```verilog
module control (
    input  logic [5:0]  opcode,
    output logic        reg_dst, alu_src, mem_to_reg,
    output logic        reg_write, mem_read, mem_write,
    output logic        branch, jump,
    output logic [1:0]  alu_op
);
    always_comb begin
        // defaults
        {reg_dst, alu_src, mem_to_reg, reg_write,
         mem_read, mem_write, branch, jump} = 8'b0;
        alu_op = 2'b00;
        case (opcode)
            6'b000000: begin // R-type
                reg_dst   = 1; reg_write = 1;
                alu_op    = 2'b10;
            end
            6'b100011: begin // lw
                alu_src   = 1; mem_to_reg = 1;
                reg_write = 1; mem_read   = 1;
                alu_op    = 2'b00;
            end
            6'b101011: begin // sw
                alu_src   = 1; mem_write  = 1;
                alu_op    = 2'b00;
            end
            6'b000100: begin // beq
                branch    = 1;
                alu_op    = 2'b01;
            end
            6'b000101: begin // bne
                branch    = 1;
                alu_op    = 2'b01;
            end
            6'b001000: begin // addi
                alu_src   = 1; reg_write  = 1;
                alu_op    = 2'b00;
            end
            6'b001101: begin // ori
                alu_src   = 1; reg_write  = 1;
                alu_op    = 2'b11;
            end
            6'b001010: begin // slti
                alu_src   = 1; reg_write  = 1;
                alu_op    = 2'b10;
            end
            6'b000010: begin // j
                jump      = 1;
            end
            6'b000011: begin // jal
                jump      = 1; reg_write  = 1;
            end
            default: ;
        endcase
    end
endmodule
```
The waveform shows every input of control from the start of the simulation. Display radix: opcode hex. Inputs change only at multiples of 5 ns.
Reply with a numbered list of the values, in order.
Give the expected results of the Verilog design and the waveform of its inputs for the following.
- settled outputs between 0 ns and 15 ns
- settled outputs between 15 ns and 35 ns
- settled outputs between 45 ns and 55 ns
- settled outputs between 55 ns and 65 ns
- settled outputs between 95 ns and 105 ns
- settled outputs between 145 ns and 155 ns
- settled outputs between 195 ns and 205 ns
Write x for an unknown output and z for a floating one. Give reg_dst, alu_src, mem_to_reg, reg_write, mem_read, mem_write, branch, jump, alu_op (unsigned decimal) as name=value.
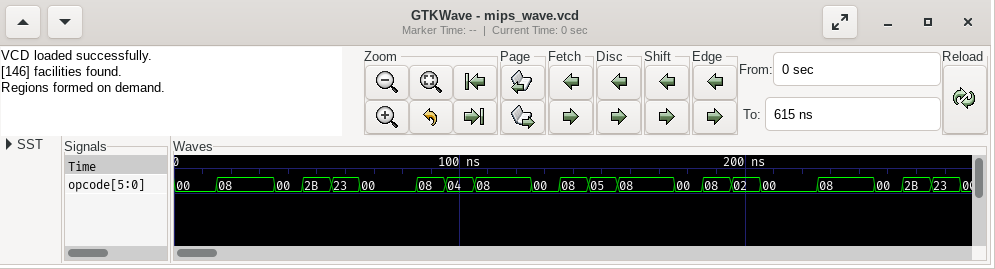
1. reg_dst=1, alu_src=0, mem_to_reg=0, reg_write=1, mem_read=0, mem_write=0, branch=0, jump=0, alu_op=2
2. reg_dst=0, alu_src=1, mem_to_reg=0, reg_write=1, mem_read=0, mem_write=0, branch=0, jump=0, alu_op=0
3. reg_dst=0, alu_src=1, mem_to_reg=0, reg_write=0, mem_read=0, mem_write=1, branch=0, jump=0, alu_op=0
4. reg_dst=0, alu_src=1, mem_to_reg=1, reg_write=1, mem_read=1, mem_write=0, branch=0, jump=0, alu_op=0
5. reg_dst=0, alu_src=0, mem_to_reg=0, reg_write=0, mem_read=0, mem_write=0, branch=1, jump=0, alu_op=1
6. reg_dst=0, alu_src=0, mem_to_reg=0, reg_write=0, mem_read=0, mem_write=0, branch=1, jump=0, alu_op=1
7. reg_dst=0, alu_src=0, mem_to_reg=0, reg_write=0, mem_read=0, mem_write=0, branch=0, jump=1, alu_op=0
